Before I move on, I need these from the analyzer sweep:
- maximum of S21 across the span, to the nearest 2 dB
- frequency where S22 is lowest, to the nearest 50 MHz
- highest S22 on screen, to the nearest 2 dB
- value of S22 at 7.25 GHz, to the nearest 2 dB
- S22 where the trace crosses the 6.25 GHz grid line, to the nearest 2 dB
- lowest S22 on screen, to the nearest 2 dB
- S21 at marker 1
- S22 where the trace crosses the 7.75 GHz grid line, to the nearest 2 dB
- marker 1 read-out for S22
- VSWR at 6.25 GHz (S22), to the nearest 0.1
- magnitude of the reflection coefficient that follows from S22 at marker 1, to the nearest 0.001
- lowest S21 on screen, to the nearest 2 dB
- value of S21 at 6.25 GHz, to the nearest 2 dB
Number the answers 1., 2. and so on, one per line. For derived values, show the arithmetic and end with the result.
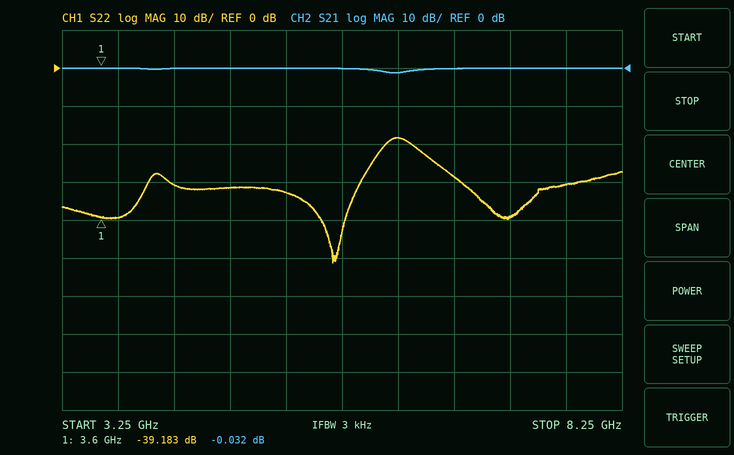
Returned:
1. 0 dB
2. 5.65 GHz
3. -18 dB
4. -40 dB
5. -18 dB
6. -52 dB
7. -0.032 dB
8. -30 dB
9. -39.183 dB
10. |Γ| = 10^(-18/20) = 0.1259; VSWR = (1 + 0.1259)/(1 − 0.1259) ≈ 1.3
11. 10^(-39.183/20) ≈ 0.011
12. -2 dB
13. -2 dB
